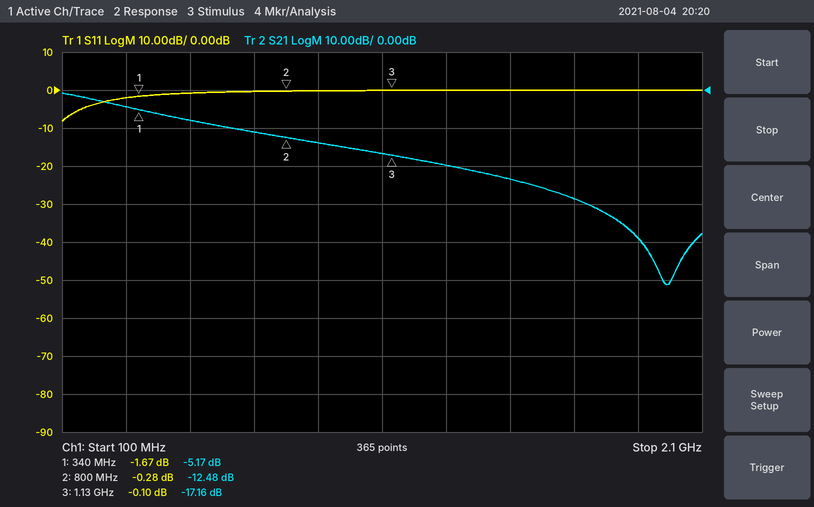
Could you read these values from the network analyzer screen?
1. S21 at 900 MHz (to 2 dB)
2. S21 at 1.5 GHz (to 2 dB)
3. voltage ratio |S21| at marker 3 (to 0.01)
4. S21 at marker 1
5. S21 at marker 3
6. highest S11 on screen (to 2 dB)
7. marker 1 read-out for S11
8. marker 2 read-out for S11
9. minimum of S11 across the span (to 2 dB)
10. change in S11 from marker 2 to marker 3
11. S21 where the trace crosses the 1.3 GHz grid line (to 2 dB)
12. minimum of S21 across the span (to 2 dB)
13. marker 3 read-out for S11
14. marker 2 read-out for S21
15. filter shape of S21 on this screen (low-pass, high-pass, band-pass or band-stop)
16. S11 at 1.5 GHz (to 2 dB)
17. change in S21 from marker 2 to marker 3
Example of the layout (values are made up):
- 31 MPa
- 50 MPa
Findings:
- -14 dB
- -24 dB
- 0.14
- -5.17 dB
- -17.16 dB
- 0 dB
- -1.67 dB
- -0.28 dB
- -8 dB
- 0.18 dB
- -20 dB
- -52 dB
- -0.10 dB
- -12.48 dB
- low-pass
- 0 dB
- -4.68 dB
